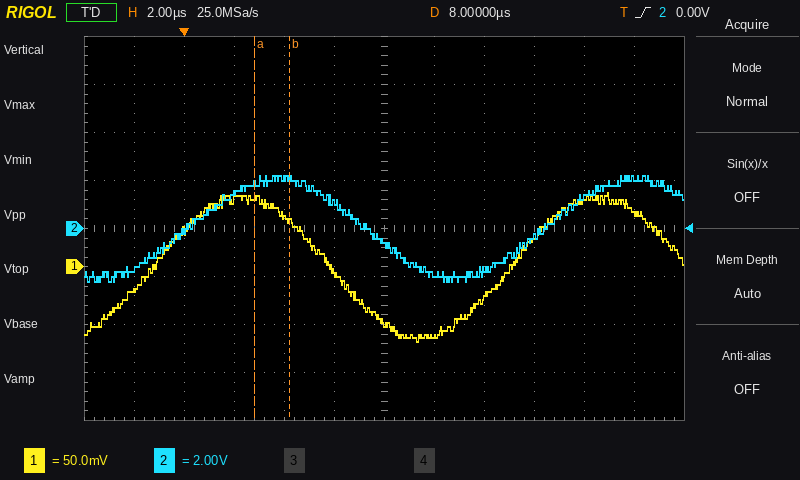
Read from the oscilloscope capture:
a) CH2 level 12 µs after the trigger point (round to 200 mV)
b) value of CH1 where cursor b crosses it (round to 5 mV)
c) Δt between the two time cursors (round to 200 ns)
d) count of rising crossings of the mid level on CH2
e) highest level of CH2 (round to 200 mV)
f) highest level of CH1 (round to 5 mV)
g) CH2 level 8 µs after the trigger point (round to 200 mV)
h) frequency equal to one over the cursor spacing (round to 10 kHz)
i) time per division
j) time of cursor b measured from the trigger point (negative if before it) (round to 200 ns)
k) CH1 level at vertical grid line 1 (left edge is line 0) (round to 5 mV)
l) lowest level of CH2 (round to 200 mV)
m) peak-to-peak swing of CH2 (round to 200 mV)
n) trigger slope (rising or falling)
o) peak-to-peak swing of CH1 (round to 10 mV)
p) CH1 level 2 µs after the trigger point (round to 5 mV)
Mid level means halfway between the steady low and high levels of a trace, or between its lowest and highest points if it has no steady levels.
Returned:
-1.8 V
45 mV
1.4 µs
2
2.2 V
80 mV
-600 mV
710 kHz
2 µs
+4.2 µs
-25 mV
-2.2 V
4.4 V
rising
160 mV
70 mV
